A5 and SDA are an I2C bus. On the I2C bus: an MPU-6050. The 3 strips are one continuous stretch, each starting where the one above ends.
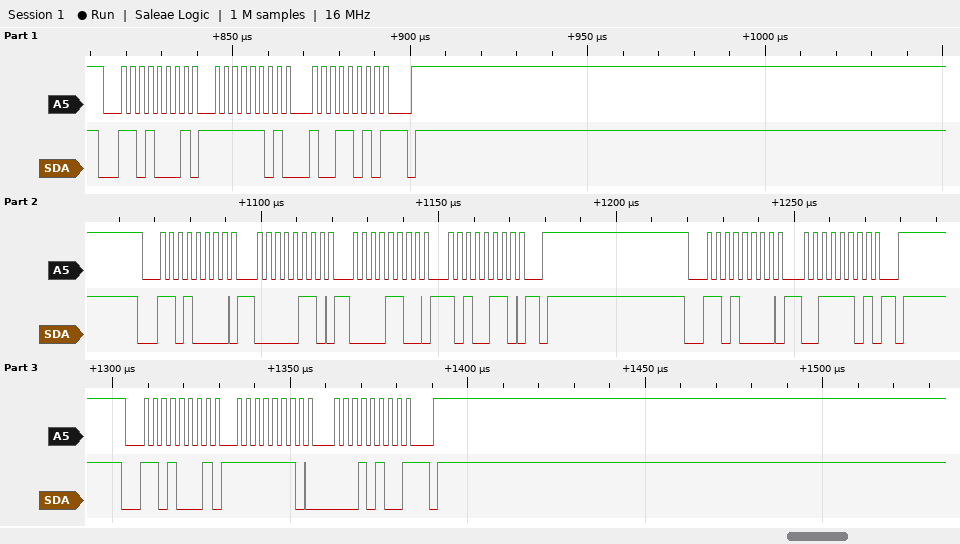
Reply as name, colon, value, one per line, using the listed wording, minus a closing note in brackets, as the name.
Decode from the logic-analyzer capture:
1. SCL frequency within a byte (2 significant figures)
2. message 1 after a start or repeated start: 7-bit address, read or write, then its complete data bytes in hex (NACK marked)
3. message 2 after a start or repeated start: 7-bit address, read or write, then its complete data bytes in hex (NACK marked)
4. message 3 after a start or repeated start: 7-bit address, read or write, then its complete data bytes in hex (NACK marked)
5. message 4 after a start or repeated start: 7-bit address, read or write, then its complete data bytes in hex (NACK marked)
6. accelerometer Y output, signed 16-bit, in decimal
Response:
SCL frequency within a byte: 400 kHz
message 1 after a start or repeated start: 7-bit address, read or write, then its complete data bytes in hex: 0x68 read: FD 9A NACK
message 2 after a start or repeated start: 7-bit address, read or write, then its complete data bytes in hex: 0x68 write: 06 0C A6
message 3 after a start or repeated start: 7-bit address, read or write, then its complete data bytes in hex: 0x68 write: 3D
message 4 after a start or repeated start: 7-bit address, read or write, then its complete data bytes in hex: 0x68 read: FE 14 NACK
accelerometer Y output, signed 16-bit, in decimal: -492
